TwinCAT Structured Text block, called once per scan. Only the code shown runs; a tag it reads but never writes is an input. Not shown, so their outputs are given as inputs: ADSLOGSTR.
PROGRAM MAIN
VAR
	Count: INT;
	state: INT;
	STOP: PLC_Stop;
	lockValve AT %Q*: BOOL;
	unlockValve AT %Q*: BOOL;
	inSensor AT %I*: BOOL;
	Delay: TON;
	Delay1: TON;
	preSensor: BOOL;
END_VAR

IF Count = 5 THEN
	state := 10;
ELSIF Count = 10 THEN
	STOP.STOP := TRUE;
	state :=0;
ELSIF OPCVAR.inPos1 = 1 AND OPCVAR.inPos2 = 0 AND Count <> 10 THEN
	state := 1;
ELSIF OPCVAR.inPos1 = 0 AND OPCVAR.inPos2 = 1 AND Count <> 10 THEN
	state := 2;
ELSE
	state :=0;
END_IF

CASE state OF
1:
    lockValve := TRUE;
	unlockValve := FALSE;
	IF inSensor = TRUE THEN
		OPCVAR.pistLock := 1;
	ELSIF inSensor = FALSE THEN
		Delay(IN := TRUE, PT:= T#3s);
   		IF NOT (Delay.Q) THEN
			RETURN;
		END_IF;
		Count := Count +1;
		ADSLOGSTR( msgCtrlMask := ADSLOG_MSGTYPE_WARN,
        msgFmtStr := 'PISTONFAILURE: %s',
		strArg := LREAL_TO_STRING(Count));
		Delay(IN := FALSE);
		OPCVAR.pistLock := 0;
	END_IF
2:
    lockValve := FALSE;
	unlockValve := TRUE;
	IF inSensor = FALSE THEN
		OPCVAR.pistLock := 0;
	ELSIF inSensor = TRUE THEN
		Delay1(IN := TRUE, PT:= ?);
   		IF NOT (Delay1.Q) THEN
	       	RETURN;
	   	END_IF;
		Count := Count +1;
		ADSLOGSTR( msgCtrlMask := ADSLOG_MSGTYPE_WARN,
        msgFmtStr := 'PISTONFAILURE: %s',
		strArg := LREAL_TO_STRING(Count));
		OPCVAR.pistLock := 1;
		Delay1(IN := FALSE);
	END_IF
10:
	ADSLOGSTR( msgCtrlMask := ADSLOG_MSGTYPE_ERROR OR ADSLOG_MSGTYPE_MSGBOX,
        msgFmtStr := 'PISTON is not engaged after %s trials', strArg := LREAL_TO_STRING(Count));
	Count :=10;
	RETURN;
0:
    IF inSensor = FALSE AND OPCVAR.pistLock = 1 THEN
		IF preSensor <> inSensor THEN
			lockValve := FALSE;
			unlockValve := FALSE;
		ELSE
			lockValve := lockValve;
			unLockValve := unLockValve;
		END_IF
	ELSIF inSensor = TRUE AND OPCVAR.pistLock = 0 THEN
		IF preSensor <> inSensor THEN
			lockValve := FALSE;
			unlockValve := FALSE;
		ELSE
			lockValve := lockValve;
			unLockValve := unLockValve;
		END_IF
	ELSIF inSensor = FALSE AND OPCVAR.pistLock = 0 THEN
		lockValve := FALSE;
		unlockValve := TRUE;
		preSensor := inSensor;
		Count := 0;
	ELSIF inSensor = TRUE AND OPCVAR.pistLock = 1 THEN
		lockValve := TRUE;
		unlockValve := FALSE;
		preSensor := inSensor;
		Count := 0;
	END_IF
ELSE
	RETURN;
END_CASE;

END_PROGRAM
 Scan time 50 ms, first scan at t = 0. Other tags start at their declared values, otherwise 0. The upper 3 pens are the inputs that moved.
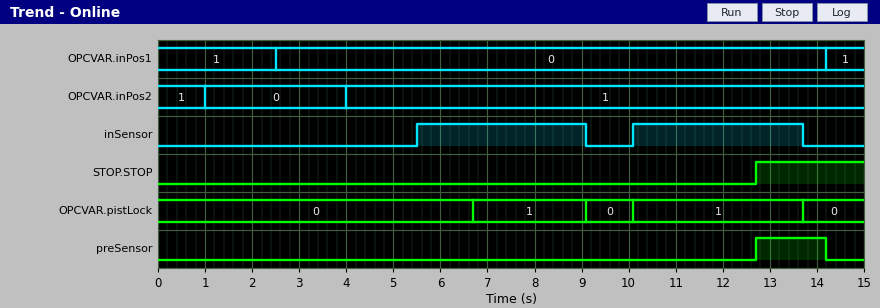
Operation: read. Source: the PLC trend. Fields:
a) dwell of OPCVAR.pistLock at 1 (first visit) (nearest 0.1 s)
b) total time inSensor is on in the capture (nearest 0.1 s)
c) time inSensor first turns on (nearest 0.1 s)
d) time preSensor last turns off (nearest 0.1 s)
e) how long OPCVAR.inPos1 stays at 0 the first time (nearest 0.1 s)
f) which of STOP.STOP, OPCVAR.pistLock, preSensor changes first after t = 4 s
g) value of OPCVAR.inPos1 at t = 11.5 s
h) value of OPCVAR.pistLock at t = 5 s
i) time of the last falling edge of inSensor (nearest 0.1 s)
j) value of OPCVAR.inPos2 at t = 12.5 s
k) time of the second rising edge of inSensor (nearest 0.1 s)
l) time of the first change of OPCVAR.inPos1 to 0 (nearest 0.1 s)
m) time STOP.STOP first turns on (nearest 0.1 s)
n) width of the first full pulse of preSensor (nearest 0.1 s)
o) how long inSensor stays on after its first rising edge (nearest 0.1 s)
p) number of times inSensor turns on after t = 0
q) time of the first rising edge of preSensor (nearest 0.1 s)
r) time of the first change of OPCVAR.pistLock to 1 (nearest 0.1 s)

2.4 s
7.2 s
5.5 s
14.2 s
11.7 s
OPCVAR.pistLock
0
0
13.7 s
1
10.1 s
2.5 s
12.7 s
1.5 s
3.6 s
2
12.7 s
6.7 s
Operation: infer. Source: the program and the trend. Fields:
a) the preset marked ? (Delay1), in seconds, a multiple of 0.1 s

1.2 s
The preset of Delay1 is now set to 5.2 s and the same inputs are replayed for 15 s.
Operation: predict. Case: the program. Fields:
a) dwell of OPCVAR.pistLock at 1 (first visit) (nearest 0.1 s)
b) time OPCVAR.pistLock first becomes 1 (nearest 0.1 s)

3.0 s
10.7 s
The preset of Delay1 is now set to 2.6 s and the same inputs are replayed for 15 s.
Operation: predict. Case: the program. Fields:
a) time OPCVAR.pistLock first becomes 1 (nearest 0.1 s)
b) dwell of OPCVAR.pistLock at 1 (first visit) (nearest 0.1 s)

8.1 s
1.0 s
